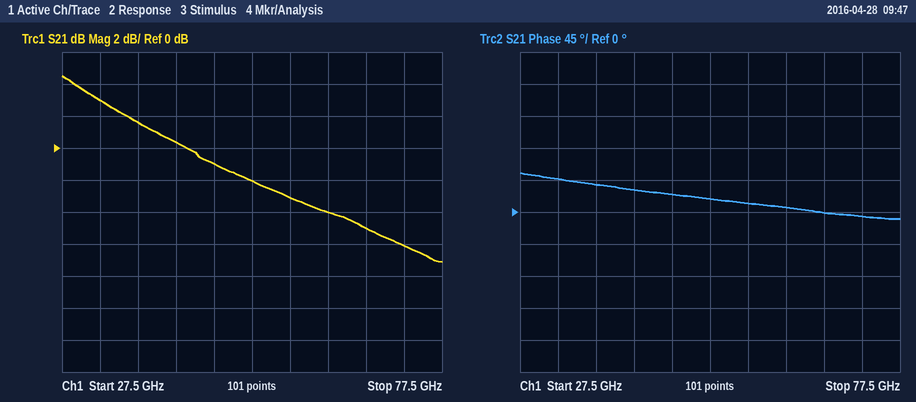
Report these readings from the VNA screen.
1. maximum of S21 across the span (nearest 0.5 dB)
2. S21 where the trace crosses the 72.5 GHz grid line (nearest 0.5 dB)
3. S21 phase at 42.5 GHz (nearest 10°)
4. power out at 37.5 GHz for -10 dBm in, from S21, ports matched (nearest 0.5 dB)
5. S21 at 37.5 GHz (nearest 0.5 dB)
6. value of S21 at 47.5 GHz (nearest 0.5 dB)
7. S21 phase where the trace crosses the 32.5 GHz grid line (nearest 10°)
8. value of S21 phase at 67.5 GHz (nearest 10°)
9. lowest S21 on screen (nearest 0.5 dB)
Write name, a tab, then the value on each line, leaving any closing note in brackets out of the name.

maximum of S21 across the span	4.5 dB
S21 where the trace crosses the 72.5 GHz grid line	-6.0 dB
S21 phase at 42.5 GHz	30°
power out at 37.5 GHz for -10 dBm in, from S21, ports matched	-8.5 dBm
S21 at 37.5 GHz	1.5 dB
value of S21 at 47.5 GHz	-1.0 dB
S21 phase where the trace crosses the 32.5 GHz grid line	50°
value of S21 phase at 67.5 GHz	0°
lowest S21 on screen	-7.0 dB
